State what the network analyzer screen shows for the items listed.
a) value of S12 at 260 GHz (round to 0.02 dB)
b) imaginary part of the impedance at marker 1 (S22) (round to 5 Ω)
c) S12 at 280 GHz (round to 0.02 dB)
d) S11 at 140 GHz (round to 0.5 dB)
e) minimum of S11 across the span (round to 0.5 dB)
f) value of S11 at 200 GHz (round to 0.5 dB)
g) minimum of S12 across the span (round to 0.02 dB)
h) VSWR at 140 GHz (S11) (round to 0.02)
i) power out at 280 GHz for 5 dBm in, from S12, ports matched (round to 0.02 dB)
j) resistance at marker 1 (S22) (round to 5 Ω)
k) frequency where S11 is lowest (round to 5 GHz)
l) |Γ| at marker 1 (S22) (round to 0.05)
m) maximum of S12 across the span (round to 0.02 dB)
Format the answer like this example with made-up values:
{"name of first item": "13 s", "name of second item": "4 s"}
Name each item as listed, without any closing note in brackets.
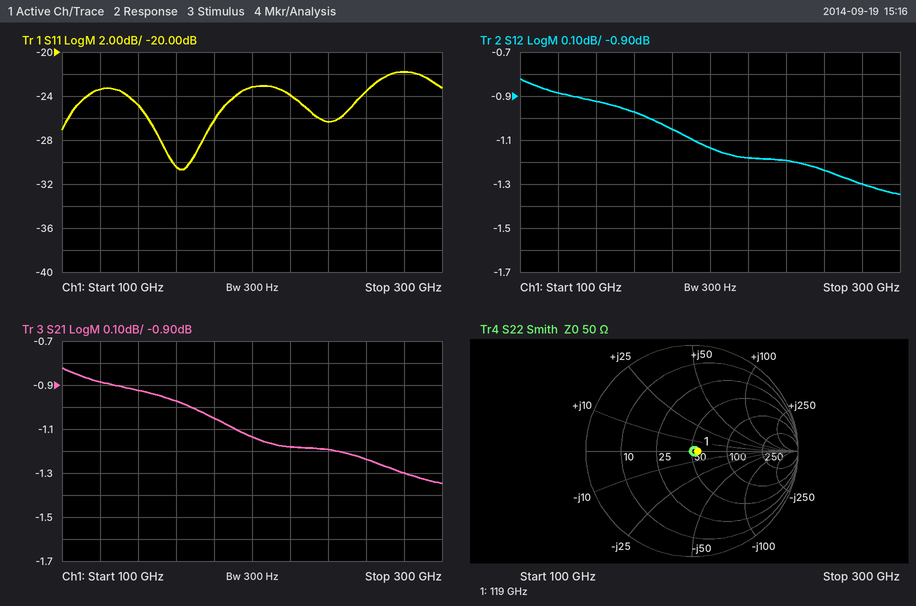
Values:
{"value of S12 at 260 GHz": "-1.24 dB", "imaginary part of the impedance at marker 1 (S22)": "0 Ω", "S12 at 280 GHz": "-1.30 dB", "S11 at 140 GHz": "-25.0 dB", "minimum of S11 across the span": "-30.5 dB", "value of S11 at 200 GHz": "-23.0 dB", "minimum of S12 across the span": "-1.34 dB", "VSWR at 140 GHz (S11)": "1.12", "power out at 280 GHz for 5 dBm in, from S12, ports matched": "3.70 dBm", "resistance at marker 1 (S22)": "55 Ω", "frequency where S11 is lowest": "160 GHz", "|Γ| at marker 1 (S22)": "0.05", "maximum of S12 across the span": "-0.82 dB"}
